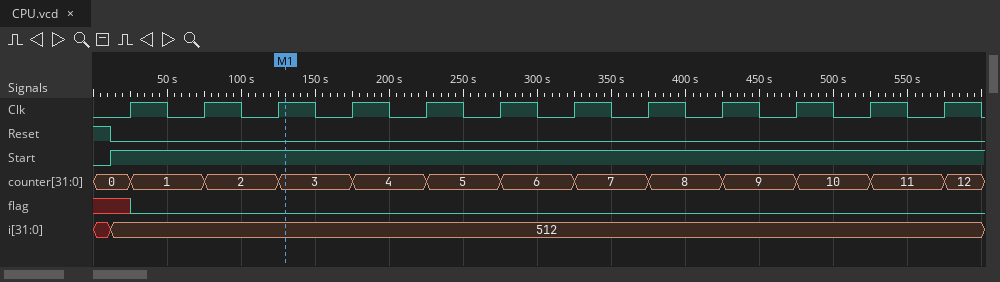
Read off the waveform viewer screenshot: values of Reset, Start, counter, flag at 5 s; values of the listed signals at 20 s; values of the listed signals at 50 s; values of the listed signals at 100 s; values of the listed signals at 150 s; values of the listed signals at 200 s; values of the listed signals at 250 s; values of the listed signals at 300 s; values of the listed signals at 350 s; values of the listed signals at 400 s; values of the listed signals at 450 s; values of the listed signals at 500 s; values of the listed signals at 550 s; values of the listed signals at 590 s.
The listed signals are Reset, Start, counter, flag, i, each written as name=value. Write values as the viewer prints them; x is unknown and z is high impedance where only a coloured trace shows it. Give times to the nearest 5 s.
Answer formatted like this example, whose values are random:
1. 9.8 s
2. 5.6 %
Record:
1. Reset=1, Start=0, counter=0, flag=x
2. Reset=0, Start=1, counter=0, flag=x, i=512
3. Reset=0, Start=1, counter=1, flag=0, i=512
4. Reset=0, Start=1, counter=2, flag=0, i=512
5. Reset=0, Start=1, counter=3, flag=0, i=512
6. Reset=0, Start=1, counter=4, flag=0, i=512
7. Reset=0, Start=1, counter=5, flag=0, i=512
8. Reset=0, Start=1, counter=6, flag=0, i=512
9. Reset=0, Start=1, counter=7, flag=0, i=512
10. Reset=0, Start=1, counter=8, flag=0, i=512
11. Reset=0, Start=1, counter=9, flag=0, i=512
12. Reset=0, Start=1, counter=10, flag=0, i=512
13. Reset=0, Start=1, counter=11, flag=0, i=512
14. Reset=0, Start=1, counter=12, flag=0, i=512
